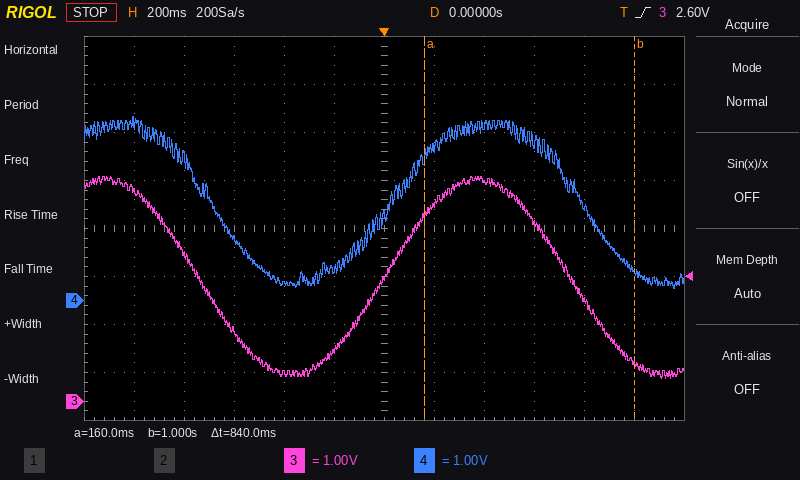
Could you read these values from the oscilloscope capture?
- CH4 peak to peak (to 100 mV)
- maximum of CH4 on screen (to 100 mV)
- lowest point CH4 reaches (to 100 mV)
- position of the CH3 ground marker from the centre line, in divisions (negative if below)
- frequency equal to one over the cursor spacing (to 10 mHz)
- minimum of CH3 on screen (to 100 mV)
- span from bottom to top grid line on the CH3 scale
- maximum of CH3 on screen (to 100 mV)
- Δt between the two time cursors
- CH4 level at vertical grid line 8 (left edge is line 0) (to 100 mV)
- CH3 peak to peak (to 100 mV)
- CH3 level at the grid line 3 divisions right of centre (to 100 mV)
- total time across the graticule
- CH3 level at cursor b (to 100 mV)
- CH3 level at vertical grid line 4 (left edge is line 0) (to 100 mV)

3.6 V
3.8 V
200 mV
-3.6 div
1.19 Hz
500 mV
8 V
4.7 V
840 ms
3.7 V
4.2 V
3.7 V
2.4 s
800 mV
600 mV
